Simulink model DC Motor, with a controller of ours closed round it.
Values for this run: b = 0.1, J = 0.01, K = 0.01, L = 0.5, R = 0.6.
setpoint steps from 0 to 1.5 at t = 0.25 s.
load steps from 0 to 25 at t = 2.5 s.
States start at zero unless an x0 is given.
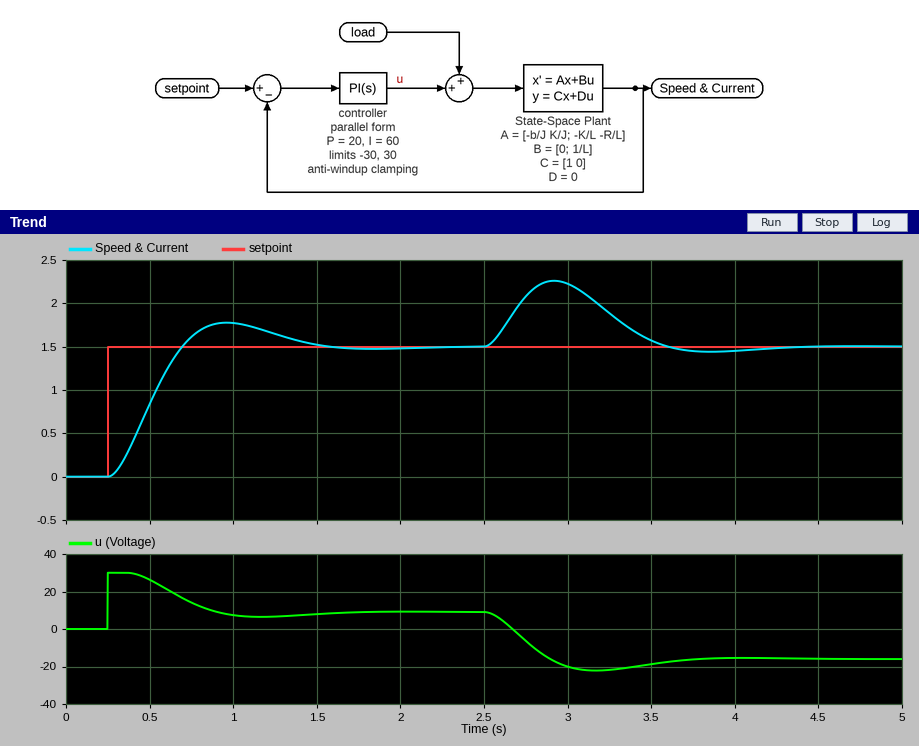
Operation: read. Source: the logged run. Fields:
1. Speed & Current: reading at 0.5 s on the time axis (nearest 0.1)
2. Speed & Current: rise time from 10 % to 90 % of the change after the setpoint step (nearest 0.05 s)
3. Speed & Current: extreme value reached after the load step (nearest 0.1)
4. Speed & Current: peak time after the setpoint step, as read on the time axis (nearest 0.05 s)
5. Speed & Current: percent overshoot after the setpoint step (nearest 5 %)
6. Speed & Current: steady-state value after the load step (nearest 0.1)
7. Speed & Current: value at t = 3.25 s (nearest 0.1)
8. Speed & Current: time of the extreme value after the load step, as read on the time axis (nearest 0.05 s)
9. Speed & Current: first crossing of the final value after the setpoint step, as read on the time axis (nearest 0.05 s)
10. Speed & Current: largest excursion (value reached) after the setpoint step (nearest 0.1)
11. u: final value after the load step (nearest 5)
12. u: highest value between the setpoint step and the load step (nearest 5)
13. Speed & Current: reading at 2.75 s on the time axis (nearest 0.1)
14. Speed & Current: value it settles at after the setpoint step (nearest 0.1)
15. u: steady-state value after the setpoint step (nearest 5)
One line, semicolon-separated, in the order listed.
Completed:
0.8; 0.30 s; 2.3; 0.95 s; 20 %; 1.5; 1.9; 2.90 s; 0.70 s; 1.8; -15; 30; 2.1; 1.5; 10
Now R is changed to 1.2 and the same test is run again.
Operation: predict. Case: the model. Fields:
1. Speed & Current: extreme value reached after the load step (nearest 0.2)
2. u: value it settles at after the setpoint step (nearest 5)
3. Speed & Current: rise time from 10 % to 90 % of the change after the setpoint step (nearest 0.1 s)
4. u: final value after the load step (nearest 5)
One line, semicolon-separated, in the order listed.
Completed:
2.2; 20; 0.4 s; -5
